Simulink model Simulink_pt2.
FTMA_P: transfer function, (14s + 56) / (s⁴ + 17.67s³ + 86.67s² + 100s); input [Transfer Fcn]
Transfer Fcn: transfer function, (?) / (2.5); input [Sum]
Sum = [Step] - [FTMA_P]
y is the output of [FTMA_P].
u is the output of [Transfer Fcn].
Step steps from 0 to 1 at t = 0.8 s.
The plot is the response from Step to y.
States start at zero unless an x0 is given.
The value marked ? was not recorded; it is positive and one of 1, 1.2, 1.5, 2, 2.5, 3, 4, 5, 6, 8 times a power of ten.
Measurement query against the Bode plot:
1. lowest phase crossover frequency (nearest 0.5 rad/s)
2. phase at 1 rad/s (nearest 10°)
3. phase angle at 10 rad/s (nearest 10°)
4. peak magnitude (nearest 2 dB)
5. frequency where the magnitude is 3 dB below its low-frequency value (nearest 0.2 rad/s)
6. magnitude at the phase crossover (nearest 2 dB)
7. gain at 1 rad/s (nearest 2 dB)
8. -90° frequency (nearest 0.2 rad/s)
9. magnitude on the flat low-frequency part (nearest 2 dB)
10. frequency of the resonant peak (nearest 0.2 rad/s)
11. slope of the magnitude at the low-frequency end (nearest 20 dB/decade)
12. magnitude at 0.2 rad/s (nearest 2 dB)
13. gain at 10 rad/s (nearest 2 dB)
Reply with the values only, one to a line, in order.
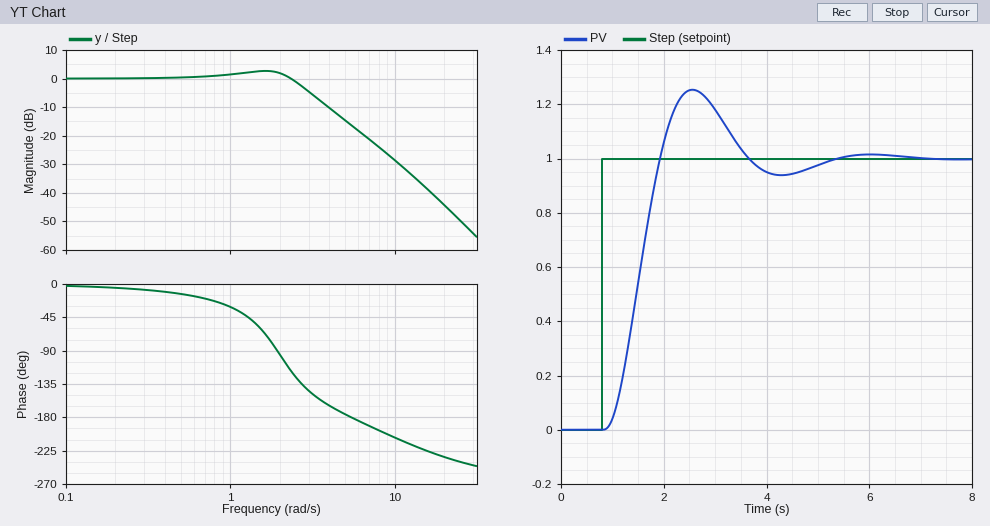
5.5 rad/s
-30°
-210°
2 dB
2.8 rad/s
-16 dB
2 dB
2.0 rad/s
0 dB
1.6 rad/s
0 dB/decade
0 dB
-28 dB
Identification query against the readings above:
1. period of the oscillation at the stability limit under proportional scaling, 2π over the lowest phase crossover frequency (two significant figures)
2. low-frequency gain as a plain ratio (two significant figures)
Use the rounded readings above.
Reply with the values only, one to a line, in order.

1.1 s
1.0
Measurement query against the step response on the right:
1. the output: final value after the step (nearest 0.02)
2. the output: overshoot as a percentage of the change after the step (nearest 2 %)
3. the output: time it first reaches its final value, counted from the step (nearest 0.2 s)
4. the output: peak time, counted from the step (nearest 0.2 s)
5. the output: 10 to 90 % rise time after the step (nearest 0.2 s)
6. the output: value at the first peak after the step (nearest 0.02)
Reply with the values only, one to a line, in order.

1.00
26 %
1.2 s
1.8 s
0.8 s
1.26
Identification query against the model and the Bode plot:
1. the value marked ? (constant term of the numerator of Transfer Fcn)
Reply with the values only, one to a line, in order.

10
